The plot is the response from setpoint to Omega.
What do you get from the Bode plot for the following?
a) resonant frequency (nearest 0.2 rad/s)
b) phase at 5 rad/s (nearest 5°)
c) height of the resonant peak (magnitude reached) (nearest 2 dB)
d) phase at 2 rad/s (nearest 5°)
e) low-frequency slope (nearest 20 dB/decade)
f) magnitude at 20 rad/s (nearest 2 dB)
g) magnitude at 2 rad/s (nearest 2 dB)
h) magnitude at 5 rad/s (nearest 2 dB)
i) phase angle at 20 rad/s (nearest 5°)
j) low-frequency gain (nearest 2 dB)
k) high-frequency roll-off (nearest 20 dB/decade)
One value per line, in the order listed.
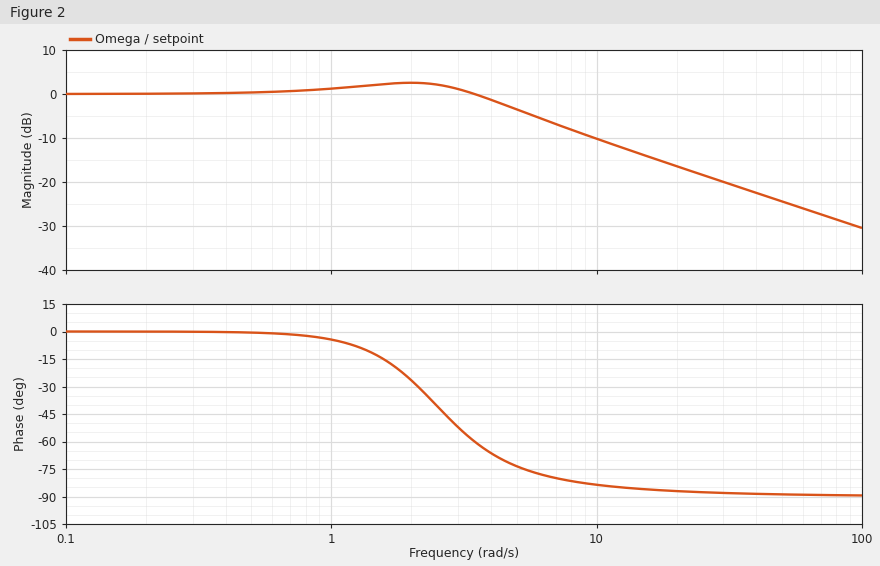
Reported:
2.0 rad/s
-75°
2 dB
-25°
0 dB/decade
-16 dB
2 dB
-4 dB
-85°
0 dB
-20 dB/decade
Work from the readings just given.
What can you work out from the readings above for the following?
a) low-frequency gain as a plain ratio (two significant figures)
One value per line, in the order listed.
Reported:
1.0
